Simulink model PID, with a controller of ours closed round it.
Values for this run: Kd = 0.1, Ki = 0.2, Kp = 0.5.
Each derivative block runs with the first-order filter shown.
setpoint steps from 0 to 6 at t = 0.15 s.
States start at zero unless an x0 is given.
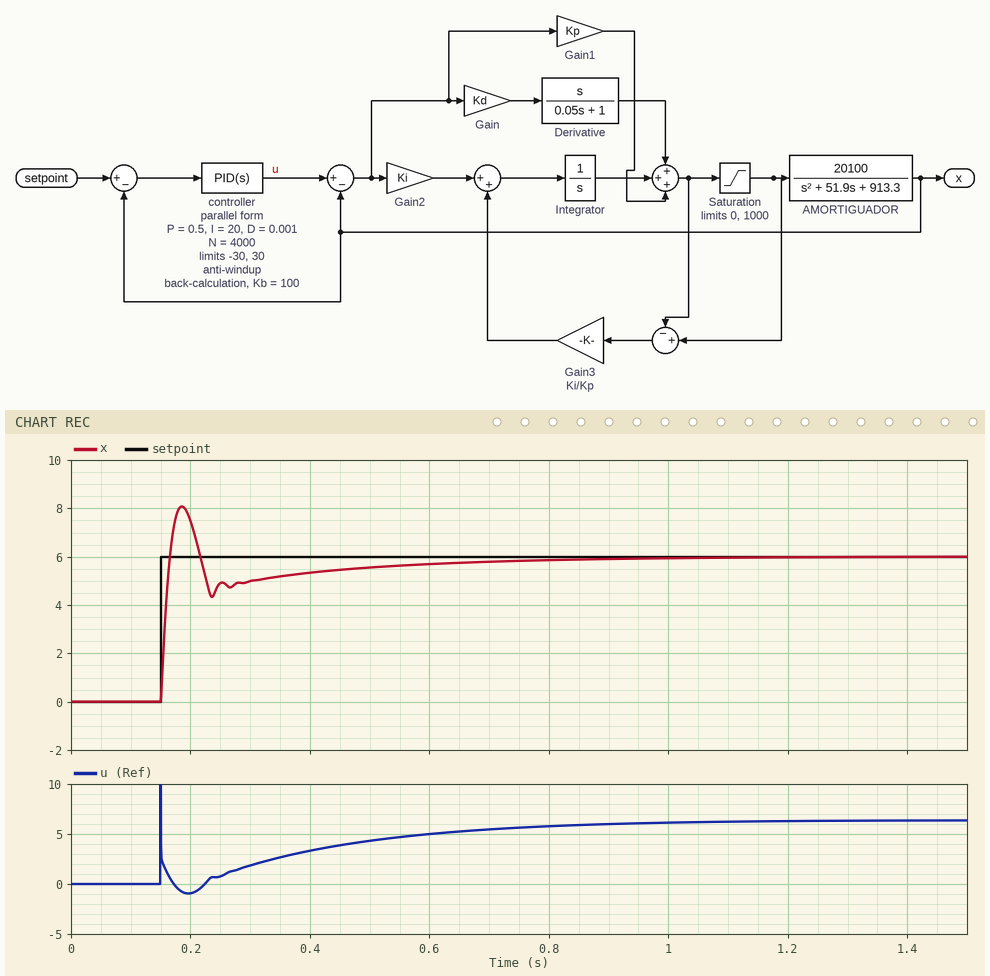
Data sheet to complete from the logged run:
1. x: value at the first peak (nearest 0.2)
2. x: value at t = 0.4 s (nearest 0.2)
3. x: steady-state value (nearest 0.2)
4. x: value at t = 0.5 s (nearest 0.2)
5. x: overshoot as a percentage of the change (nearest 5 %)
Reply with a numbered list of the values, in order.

1. 8.0
2. 5.4
3. 6.0
4. 5.6
5. 35 %
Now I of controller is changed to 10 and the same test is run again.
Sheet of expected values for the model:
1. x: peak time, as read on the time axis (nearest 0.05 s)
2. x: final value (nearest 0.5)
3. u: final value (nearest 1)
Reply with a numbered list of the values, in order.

1. 0.20 s
2. 6.0
3. 6
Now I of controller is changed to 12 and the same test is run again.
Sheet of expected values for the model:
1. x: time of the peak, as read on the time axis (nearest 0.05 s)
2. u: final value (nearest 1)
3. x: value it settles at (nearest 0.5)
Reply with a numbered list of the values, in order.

1. 0.20 s
2. 6
3. 6.0
